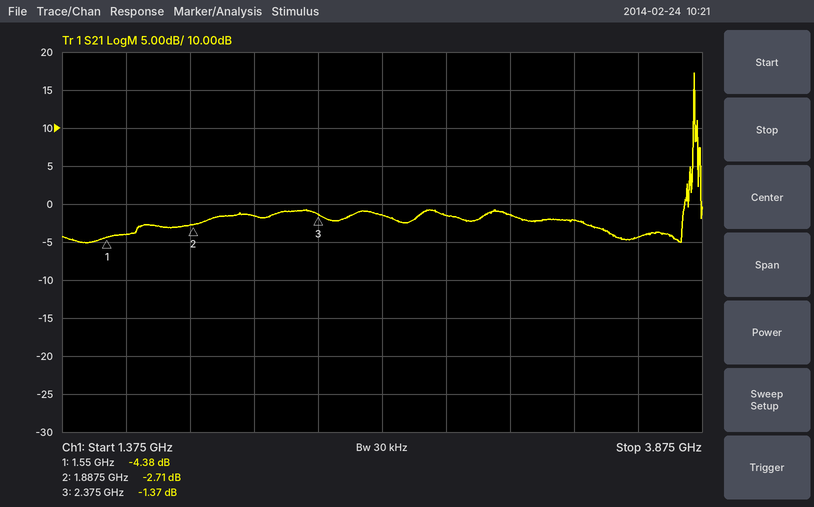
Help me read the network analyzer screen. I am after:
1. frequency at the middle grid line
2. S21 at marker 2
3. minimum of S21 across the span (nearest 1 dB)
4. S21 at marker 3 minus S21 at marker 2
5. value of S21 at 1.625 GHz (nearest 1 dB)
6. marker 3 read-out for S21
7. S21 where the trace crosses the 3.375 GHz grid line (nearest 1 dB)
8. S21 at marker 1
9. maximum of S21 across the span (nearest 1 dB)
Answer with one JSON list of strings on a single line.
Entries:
["2.625 GHz", "-2.71 dB", "-5 dB", "1.34 dB", "-4 dB", "-1.37 dB", "-2 dB", "-4.38 dB", "17 dB"]
